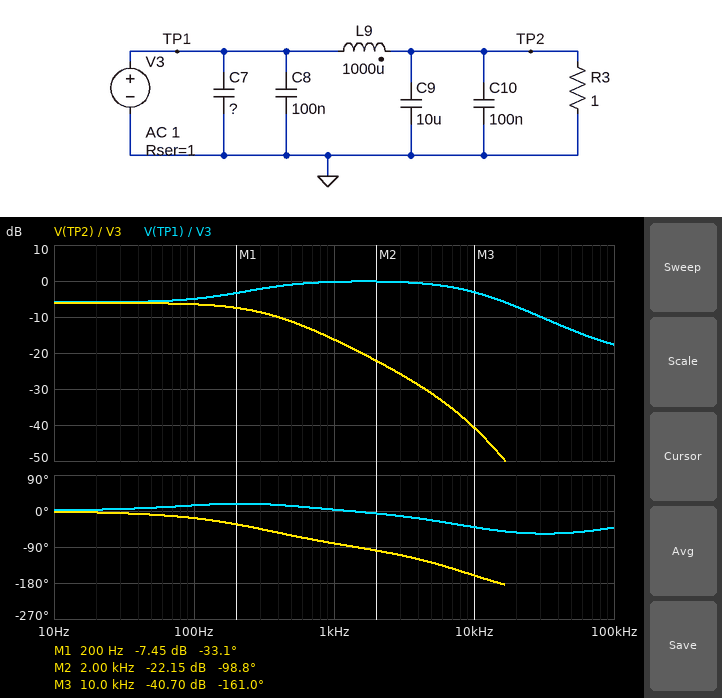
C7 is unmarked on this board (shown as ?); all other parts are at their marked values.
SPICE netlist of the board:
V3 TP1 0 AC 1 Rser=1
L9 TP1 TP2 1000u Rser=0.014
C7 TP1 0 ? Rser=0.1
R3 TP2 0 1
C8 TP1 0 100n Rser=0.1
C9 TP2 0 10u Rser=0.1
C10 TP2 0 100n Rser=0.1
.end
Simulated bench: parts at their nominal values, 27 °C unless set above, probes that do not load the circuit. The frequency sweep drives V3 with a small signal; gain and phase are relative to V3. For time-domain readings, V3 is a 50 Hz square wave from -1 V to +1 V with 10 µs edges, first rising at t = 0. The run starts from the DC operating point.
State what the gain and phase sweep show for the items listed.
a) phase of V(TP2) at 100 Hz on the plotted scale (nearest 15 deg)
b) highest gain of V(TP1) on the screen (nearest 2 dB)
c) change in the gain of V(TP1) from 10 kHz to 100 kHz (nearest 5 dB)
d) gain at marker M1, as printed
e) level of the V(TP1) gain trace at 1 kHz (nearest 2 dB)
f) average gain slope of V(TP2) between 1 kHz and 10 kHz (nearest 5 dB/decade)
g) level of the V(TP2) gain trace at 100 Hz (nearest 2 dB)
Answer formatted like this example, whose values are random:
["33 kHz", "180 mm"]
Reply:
["-15 deg", "0 dB", "-15 dB", "-7.45 dB", "0 dB", "-25 dB/decade", "-6 dB"]
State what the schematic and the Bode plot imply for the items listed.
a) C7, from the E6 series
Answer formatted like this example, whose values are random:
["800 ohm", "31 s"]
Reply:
["15 µF"]
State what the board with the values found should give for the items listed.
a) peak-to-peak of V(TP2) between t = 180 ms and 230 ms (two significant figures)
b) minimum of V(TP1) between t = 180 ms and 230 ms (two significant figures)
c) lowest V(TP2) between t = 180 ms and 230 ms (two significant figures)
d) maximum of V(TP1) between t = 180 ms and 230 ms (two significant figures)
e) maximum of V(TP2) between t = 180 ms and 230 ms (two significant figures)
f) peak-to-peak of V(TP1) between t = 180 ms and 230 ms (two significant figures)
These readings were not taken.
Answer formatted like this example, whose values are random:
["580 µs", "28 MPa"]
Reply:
["990 mV", "-1.4 V", "-500 mV", "1.4 V", "500 mV", "2.8 V"]
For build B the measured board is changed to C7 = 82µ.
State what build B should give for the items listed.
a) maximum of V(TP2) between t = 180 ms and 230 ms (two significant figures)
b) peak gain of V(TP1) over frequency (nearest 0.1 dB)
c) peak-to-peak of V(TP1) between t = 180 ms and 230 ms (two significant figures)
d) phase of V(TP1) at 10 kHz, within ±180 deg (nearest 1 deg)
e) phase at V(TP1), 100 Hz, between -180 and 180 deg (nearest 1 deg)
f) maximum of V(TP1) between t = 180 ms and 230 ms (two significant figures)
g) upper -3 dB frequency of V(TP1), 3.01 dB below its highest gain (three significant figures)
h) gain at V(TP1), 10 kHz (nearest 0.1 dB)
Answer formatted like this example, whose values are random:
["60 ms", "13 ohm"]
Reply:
["500 mV", "-0.6 dB", "2.4 V", "-53 deg", "13 deg", "1.2 V", "2.14 kHz", "-14.2 dB"]
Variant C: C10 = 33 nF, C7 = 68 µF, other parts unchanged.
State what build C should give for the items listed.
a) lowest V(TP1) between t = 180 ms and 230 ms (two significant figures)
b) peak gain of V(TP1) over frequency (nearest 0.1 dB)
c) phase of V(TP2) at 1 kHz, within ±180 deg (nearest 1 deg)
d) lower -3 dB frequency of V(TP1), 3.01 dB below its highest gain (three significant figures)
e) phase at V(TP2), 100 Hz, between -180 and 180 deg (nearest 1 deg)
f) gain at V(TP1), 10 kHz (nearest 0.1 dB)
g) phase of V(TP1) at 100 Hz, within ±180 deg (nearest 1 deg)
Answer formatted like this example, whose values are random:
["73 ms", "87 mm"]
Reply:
["-1.2 V", "-0.5 dB", "-99 deg", "181 Hz", "-19 deg", "-12.9 dB", "13 deg"]
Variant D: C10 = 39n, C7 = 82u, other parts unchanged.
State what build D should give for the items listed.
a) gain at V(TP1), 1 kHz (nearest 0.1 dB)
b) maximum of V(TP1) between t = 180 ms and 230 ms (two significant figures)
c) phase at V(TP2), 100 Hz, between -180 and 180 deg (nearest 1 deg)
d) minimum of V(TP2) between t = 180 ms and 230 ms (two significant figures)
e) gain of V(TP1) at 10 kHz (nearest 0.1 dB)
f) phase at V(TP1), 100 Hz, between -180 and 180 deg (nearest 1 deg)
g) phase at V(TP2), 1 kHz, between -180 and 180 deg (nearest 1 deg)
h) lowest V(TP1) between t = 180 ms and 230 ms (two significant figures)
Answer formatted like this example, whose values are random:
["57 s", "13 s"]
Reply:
["-0.9 dB", "1.2 V", "-19 deg", "-500 mV", "-14.2 dB", "13 deg", "-103 deg", "-1.2 V"]
